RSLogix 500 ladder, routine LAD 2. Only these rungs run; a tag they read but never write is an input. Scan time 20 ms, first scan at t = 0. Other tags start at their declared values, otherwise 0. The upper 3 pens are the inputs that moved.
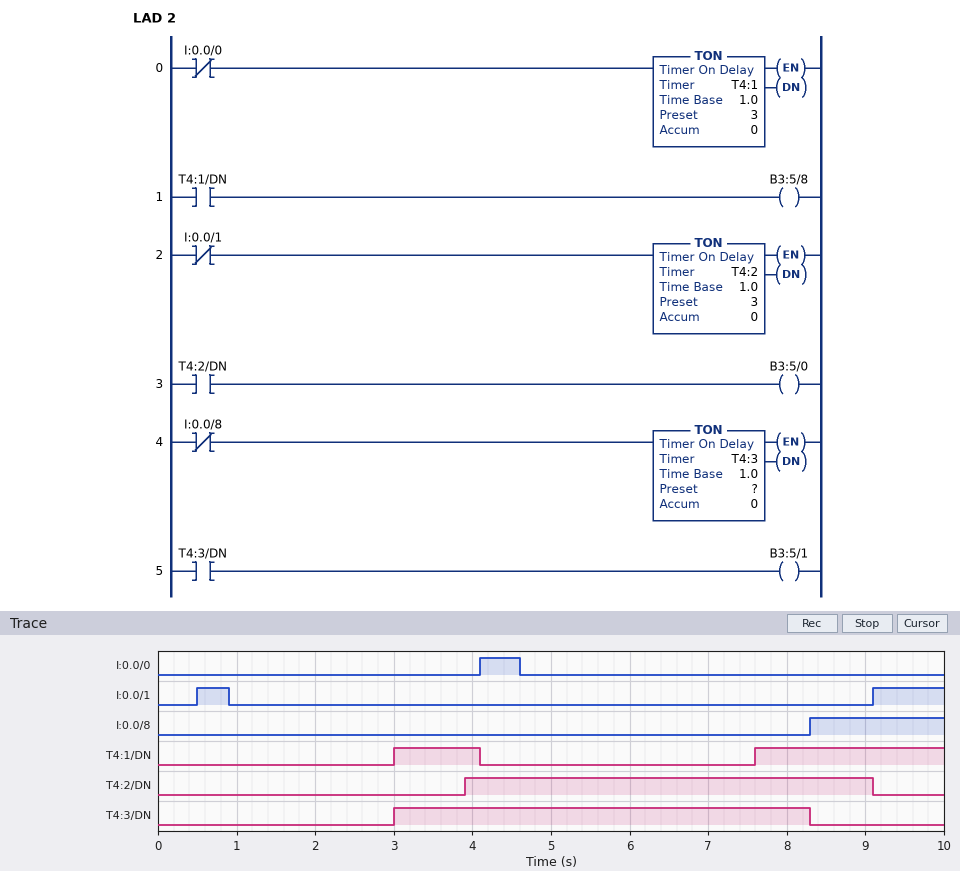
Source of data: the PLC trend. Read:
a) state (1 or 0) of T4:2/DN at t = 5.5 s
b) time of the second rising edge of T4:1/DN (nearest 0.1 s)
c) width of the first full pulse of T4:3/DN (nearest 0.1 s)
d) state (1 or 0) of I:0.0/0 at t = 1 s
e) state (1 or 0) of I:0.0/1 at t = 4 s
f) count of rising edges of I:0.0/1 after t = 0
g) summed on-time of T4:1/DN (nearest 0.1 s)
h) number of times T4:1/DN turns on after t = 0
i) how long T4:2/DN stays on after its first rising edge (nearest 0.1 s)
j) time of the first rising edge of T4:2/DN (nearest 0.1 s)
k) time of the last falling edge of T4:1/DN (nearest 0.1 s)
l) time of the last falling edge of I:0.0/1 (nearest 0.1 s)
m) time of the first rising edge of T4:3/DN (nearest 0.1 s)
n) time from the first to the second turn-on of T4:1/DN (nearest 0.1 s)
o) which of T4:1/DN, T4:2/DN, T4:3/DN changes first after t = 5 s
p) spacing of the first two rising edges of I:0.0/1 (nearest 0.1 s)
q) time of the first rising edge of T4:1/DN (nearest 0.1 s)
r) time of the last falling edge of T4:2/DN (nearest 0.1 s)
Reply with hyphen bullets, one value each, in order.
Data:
- 1
- 7.6 s
- 5.3 s
- 0
- 0
- 2
- 3.5 s
- 2
- 5.2 s
- 3.9 s
- 4.1 s
- 0.9 s
- 3.0 s
- 4.6 s
- T4:1/DN
- 8.6 s
- 3.0 s
- 9.1 s
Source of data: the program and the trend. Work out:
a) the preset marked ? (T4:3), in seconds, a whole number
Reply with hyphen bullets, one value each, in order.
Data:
- 3 s
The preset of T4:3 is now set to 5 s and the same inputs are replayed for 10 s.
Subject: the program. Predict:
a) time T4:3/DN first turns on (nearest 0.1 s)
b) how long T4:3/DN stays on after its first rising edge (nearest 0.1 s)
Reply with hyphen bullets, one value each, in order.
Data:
- 5.0 s
- 3.3 s
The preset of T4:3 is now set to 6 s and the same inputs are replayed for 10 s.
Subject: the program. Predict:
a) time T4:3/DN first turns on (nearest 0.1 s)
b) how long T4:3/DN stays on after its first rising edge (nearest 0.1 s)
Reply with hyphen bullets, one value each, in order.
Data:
- 6.0 s
- 2.3 s
